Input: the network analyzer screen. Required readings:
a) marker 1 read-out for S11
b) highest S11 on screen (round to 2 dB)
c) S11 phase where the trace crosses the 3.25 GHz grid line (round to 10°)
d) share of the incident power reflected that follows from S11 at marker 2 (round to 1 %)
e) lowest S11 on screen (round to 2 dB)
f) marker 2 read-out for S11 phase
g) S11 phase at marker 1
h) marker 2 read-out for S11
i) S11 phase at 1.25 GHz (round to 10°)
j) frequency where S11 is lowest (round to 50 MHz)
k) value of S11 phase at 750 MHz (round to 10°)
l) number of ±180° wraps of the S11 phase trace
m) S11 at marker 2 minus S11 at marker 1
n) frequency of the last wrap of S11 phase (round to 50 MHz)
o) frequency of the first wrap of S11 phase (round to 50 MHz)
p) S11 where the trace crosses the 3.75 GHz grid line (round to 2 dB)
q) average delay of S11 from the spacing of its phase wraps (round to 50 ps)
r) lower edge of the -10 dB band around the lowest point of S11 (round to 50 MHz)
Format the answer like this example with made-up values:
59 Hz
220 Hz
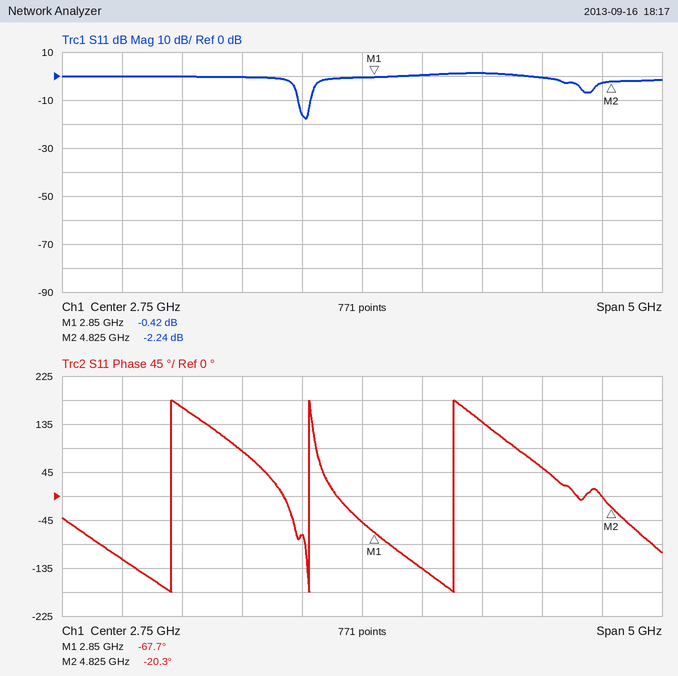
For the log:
-0.42 dB
2 dB
-140°
60 %
-18 dB
-20.3°
-67.7°
-2.24 dB
170°
2.30 GHz
-120°
3
-1.82 dB
3.50 GHz
1.15 GHz
2 dB
850 ps
2.20 GHz
